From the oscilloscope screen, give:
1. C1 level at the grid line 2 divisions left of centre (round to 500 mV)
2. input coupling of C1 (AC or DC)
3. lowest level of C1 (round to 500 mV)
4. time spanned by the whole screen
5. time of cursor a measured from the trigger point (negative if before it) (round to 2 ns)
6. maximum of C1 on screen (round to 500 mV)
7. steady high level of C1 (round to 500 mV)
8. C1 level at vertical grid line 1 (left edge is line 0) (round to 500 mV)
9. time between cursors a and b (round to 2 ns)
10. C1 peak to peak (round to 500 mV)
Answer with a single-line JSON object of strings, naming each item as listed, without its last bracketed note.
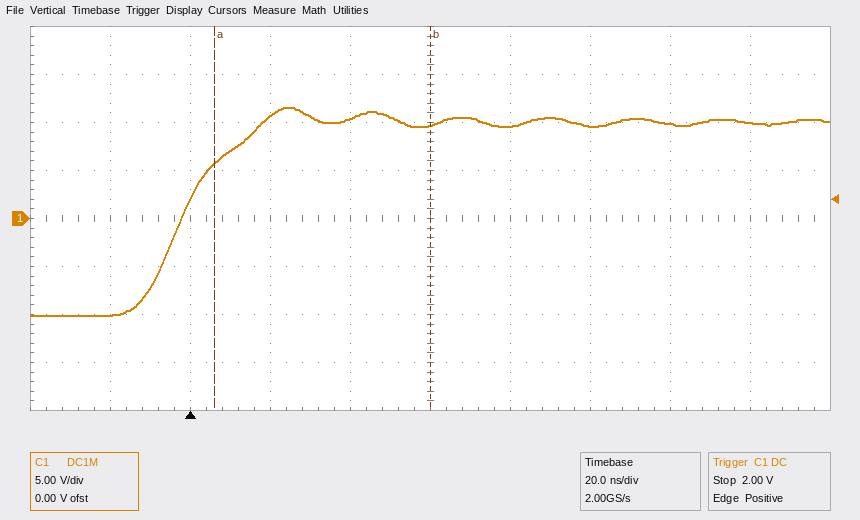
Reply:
{"C1 level at the grid line 2 divisions left of centre": "10.5 V", "input coupling of C1": "DC", "lowest level of C1": "-10.0 V", "time spanned by the whole screen": "200 ns", "time of cursor a measured from the trigger point (negative if before it)": "+6 ns", "maximum of C1 on screen": "11.5 V", "steady high level of C1": "10.0 V", "C1 level at vertical grid line 1 (left edge is line 0)": "-10.0 V", "time between cursors a and b": "54 ns", "C1 peak to peak": "21.5 V"}
